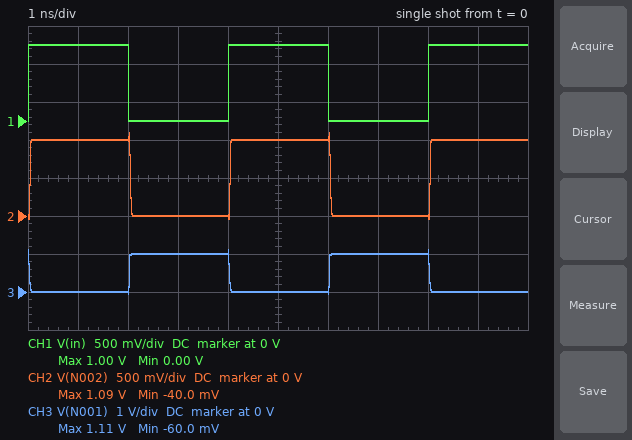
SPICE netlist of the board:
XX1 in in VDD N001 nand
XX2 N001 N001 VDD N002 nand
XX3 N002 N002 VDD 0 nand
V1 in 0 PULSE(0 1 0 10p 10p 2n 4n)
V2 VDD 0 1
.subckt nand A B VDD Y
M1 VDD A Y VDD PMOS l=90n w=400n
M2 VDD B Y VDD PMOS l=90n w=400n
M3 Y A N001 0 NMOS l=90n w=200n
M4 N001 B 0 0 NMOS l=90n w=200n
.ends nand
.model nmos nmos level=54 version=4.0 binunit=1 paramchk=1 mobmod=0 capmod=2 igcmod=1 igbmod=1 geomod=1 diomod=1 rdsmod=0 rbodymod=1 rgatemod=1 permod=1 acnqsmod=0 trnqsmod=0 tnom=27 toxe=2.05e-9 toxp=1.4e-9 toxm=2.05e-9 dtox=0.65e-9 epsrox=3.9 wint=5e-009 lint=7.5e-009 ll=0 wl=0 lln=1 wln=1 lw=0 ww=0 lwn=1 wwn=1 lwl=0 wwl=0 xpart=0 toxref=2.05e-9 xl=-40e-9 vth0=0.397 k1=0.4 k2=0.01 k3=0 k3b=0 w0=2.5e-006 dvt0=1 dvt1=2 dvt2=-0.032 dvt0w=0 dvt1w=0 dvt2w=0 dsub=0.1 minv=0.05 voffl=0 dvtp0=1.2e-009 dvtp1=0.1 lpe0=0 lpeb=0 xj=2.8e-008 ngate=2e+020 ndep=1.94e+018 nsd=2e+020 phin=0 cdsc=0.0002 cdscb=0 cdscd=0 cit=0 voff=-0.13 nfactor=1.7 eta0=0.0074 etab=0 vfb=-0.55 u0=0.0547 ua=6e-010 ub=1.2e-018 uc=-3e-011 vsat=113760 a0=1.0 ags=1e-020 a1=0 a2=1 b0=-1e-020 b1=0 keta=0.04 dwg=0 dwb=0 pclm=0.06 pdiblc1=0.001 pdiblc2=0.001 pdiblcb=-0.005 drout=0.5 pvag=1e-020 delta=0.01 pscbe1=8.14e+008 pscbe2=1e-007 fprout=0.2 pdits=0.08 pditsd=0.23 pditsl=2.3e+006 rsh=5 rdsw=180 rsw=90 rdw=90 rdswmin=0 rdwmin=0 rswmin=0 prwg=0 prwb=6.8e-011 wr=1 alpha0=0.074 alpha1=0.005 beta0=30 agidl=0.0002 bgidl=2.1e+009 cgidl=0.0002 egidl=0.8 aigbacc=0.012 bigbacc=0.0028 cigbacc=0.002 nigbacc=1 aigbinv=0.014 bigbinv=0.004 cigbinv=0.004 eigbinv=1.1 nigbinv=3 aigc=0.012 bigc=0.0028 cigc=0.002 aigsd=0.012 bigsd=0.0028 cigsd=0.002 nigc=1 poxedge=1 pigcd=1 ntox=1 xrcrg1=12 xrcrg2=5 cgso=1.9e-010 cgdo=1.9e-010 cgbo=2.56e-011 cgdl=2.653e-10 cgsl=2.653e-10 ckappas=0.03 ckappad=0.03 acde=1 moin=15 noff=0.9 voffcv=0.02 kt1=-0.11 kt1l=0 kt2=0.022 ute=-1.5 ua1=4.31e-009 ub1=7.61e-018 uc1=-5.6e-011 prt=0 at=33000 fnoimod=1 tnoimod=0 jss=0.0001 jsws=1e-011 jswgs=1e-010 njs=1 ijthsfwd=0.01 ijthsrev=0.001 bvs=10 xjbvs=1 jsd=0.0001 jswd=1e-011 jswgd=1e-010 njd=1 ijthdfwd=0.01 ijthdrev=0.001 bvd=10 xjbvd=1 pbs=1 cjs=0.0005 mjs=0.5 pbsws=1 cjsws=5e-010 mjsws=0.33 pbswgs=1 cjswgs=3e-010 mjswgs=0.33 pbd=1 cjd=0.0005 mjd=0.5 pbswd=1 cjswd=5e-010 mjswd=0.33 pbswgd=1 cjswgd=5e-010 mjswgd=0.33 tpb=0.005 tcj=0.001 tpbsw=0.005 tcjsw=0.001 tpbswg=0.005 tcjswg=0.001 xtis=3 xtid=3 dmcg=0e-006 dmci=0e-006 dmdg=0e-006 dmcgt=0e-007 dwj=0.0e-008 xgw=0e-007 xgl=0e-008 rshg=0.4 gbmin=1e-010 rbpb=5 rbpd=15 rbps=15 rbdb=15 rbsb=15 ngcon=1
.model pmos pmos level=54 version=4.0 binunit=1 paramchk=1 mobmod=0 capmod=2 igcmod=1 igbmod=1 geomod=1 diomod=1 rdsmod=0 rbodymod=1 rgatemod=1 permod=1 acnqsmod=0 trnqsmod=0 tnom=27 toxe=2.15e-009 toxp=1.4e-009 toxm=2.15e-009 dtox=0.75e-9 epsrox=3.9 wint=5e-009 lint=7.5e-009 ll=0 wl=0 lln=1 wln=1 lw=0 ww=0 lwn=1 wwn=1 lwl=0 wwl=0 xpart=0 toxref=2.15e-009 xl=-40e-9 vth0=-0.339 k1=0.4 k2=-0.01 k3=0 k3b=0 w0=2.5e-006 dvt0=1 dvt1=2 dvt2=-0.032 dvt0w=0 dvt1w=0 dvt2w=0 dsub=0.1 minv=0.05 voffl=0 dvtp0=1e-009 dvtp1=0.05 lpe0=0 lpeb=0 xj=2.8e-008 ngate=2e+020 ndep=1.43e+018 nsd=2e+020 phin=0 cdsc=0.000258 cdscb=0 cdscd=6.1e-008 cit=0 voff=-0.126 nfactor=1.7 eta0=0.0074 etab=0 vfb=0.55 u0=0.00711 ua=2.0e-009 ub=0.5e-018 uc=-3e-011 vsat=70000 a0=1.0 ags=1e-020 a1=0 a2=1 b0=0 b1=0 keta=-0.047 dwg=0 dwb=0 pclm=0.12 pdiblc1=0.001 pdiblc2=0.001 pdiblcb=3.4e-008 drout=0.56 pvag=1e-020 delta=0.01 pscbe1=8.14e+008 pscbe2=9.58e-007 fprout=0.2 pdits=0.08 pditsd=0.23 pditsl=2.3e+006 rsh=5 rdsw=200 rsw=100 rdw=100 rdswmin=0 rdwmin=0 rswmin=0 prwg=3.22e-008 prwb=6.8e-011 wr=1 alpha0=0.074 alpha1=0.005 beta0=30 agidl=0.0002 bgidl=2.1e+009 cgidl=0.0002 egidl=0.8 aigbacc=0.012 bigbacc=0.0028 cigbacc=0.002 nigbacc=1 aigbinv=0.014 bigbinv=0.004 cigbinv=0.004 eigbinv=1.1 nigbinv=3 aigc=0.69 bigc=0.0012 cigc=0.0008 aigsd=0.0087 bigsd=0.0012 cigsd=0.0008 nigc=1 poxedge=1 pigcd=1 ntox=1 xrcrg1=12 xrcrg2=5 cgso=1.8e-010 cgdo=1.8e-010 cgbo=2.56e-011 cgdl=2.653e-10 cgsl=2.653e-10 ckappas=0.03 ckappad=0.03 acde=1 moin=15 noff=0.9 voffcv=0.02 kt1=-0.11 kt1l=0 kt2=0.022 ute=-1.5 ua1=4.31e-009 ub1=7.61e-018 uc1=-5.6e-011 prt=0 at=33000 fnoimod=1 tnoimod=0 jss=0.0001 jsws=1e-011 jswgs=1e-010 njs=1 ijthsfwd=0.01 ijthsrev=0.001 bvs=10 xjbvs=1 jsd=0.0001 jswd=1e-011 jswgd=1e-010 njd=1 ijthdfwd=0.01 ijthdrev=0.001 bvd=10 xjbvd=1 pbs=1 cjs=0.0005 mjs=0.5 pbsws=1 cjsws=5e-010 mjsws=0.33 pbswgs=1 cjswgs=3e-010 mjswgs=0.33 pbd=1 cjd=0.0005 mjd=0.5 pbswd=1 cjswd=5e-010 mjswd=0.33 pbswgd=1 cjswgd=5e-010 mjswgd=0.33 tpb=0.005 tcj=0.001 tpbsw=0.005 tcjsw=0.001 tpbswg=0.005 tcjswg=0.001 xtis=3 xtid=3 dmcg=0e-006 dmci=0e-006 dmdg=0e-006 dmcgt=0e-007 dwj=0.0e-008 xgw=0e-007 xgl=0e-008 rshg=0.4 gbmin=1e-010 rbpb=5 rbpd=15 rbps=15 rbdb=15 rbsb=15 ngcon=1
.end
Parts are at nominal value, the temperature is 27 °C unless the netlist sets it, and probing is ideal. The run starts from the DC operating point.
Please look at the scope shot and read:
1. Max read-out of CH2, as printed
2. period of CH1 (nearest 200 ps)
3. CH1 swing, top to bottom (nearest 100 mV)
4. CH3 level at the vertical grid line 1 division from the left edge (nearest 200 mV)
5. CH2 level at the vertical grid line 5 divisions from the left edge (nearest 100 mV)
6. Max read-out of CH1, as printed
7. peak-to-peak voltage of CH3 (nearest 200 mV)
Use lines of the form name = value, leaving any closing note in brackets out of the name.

Max read-out of CH2, as printed = 1.09 V
period of CH1 = 4.0 ns
CH1 swing, top to bottom = 1.0 V
CH3 level at the vertical grid line 1 division from the left edge = 0 V
CH2 level at the vertical grid line 5 divisions from the left edge = 1.0 V
Max read-out of CH1, as printed = 1.00 V
peak-to-peak voltage of CH3 = 1.2 V
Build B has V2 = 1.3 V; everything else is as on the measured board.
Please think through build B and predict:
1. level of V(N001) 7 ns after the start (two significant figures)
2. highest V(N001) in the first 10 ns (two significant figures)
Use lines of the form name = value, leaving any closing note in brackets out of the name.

level of V(N001) 7 ns after the start = 1.3 V
highest V(N001) in the first 10 ns = 1.4 V
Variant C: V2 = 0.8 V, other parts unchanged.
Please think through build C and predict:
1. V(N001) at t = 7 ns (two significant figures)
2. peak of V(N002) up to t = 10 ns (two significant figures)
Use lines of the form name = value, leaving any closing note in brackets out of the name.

V(N001) at t = 7 ns = 800 mV
peak of V(N002) up to t = 10 ns = 890 mV
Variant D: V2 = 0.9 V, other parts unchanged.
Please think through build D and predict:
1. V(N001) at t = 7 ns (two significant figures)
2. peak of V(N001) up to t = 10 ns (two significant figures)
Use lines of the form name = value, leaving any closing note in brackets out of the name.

V(N001) at t = 7 ns = 900 mV
peak of V(N001) up to t = 10 ns = 1.0 V
